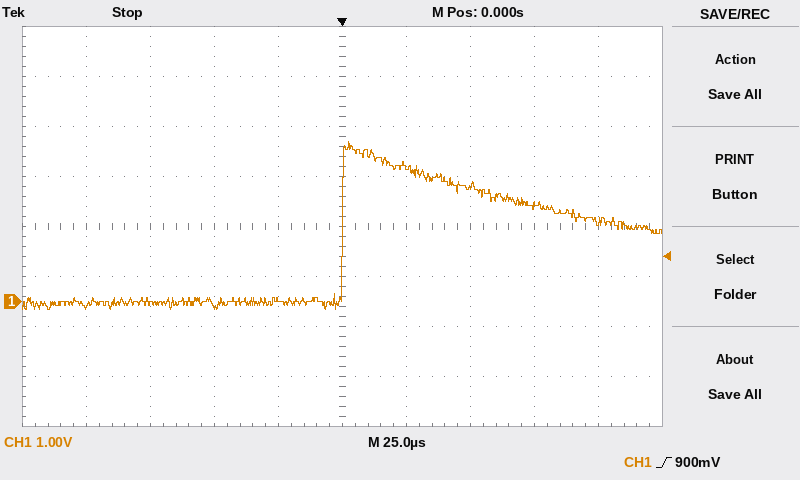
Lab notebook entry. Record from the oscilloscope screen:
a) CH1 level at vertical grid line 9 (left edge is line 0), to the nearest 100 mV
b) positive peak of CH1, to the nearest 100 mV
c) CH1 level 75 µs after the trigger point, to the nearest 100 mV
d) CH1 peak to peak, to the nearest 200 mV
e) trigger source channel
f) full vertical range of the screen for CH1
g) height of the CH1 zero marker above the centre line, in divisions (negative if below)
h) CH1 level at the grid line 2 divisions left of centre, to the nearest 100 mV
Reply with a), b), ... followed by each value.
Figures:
a) 1.6 V
b) 3.2 V
c) 1.9 V
d) 3.4 V
e) CH1
f) 8 V
g) -1.5 div
h) -100 mV
